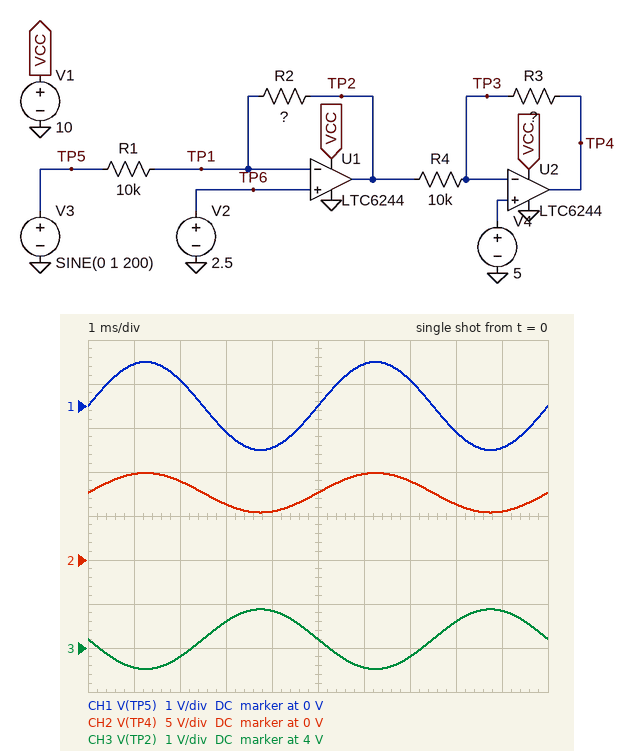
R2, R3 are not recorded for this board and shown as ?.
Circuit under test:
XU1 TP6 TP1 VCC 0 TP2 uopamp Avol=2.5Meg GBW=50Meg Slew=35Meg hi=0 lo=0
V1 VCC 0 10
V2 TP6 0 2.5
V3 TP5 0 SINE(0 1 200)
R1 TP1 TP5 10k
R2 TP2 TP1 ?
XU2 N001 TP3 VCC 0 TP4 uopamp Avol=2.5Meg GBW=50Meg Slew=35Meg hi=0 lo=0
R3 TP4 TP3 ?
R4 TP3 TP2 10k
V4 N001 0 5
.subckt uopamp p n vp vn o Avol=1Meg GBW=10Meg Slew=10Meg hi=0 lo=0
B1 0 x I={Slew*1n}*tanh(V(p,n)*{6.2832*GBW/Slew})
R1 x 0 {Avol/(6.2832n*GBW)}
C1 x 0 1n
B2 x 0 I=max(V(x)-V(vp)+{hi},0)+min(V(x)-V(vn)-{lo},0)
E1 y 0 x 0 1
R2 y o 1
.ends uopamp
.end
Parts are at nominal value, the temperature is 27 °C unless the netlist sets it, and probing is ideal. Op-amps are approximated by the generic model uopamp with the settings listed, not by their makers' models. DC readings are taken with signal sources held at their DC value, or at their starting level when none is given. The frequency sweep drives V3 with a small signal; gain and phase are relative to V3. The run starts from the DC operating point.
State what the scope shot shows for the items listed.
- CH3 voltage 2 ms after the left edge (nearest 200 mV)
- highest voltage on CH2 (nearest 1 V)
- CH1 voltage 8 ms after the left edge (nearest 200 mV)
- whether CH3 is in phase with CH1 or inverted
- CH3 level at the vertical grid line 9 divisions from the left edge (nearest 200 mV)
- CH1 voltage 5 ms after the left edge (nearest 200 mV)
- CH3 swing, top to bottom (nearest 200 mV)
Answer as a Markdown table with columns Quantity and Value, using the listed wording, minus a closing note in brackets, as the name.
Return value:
| Quantity | Value |
|---|---|
| CH3 voltage 2 ms after the left edge | 3.8 V |
| highest voltage on CH2 | 10 V |
| CH1 voltage 8 ms after the left edge | -600 mV |
| whether CH3 is in phase with CH1 or inverted | inverted |
| CH3 level at the vertical grid line 9 divisions from the left edge | 4.8 V |
| CH1 voltage 5 ms after the left edge | 0 V |
| CH3 swing, top to bottom | 1.4 V |
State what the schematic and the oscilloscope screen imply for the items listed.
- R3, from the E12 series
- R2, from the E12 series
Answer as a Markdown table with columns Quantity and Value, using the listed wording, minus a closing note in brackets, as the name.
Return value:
| Quantity | Value |
|---|---|
| R3, from the E12 series | 33 kΩ |
| R2, from the E12 series | 6.8 kΩ |
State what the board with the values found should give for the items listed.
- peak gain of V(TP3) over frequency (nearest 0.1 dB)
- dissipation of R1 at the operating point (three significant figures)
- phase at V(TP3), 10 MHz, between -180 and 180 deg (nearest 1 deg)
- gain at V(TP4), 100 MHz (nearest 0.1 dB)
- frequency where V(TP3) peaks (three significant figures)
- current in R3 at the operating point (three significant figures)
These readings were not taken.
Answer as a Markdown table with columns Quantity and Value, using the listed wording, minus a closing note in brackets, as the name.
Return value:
| Quantity | Value |
|---|---|
| peak gain of V(TP3) over frequency | -8.5 dB |
| dissipation of R1 at the operating point | 625 µW |
| phase at V(TP3), 10 MHz, between -180 and 180 deg | -149 deg |
| gain at V(TP4), 100 MHz | -22.6 dB |
| frequency where V(TP3) peaks | 18.6 MHz |
| current in R3 at the operating point | 80.0 µA |
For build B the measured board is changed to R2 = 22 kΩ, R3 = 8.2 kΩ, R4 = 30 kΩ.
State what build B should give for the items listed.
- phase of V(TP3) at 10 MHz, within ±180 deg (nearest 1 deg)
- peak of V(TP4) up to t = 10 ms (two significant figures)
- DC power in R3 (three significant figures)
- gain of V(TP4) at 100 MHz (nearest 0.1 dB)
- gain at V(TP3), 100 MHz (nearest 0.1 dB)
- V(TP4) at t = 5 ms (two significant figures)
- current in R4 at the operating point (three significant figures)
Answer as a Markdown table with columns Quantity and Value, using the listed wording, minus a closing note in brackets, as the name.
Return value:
| Quantity | Value |
|---|---|
| phase of V(TP3) at 10 MHz, within ±180 deg | -137 deg |
| peak of V(TP4) up to t = 10 ms | 4.8 V |
| DC power in R3 | 82.0 µW |
| gain of V(TP4) at 100 MHz | -29.4 dB |
| gain at V(TP3), 100 MHz | -23.4 dB |
| V(TP4) at t = 5 ms | 4.2 V |
| current in R4 at the operating point | 100 µA |
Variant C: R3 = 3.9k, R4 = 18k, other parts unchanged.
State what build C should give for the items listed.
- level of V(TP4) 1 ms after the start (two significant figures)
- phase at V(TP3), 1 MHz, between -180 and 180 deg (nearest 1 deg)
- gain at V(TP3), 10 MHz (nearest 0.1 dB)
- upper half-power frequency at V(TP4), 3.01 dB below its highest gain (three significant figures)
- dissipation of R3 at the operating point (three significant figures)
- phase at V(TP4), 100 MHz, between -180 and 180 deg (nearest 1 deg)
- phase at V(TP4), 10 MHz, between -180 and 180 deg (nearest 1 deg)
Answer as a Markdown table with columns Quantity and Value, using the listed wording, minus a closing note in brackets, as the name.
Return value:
| Quantity | Value |
|---|---|
| level of V(TP4) 1 ms after the start | 5.3 V |
| phase at V(TP3), 1 MHz, between -180 and 180 deg | -93 deg |
| gain at V(TP3), 10 MHz | -31.3 dB |
| upper half-power frequency at V(TP4), 3.01 dB below its highest gain | 22.1 MHz |
| dissipation of R3 at the operating point | 7.70 µW |
| phase at V(TP4), 100 MHz, between -180 and 180 deg | -141 deg |
| phase at V(TP4), 10 MHz, between -180 and 180 deg | -32 deg |
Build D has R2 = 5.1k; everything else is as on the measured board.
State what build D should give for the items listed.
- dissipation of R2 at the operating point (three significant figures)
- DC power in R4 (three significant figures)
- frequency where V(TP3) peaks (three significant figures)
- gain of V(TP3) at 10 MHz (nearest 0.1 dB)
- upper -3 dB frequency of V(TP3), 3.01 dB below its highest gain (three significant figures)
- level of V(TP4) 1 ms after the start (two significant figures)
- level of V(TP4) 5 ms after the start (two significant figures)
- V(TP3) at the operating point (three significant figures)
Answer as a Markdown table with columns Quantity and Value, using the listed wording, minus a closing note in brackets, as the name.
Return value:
| Quantity | Value |
|---|---|
| dissipation of R2 at the operating point | 319 µW |
| DC power in R4 | 150 µW |
| frequency where V(TP3) peaks | 19.6 MHz |
| gain of V(TP3) at 10 MHz | -12.2 dB |
| upper -3 dB frequency of V(TP3), 3.01 dB below its highest gain | 52.1 MHz |
| level of V(TP4) 1 ms after the start | 10 V |
| level of V(TP4) 5 ms after the start | 9.0 V |
| V(TP3) at the operating point | 5.00 V |
